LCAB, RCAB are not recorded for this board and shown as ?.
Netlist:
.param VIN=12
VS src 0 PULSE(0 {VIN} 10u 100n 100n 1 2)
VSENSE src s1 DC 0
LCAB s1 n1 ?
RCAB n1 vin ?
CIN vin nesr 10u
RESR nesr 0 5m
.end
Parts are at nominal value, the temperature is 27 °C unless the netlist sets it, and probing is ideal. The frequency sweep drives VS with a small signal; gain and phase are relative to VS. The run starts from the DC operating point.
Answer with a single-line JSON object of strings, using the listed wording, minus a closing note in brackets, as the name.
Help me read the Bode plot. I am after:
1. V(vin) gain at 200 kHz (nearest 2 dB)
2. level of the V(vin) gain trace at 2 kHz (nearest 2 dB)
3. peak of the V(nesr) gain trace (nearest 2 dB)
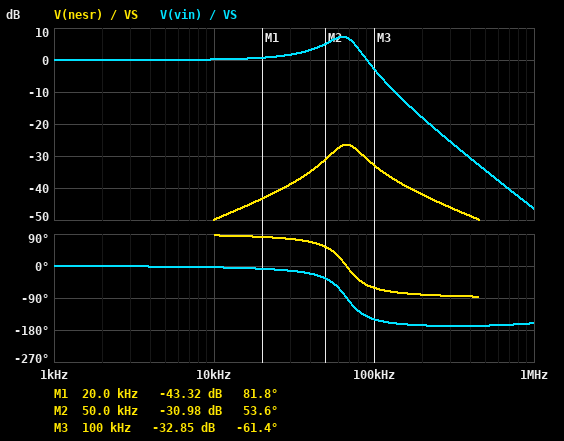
{"V(vin) gain at 200 kHz": "-18 dB", "level of the V(vin) gain trace at 2 kHz": "0 dB", "peak of the V(nesr) gain trace": "-26 dB"}
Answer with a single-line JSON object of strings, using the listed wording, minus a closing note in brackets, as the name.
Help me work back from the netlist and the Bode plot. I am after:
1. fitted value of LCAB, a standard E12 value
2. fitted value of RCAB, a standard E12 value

{"fitted value of LCAB, a standard E12 value": "560 nH", "fitted value of RCAB, a standard E12 value": "0.1 Ω"}
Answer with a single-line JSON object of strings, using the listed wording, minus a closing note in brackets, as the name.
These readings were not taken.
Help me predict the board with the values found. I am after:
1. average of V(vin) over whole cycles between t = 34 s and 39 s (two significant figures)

{"average of V(vin) over whole cycles between t = 34 s and 39 s": "6.0 V"}
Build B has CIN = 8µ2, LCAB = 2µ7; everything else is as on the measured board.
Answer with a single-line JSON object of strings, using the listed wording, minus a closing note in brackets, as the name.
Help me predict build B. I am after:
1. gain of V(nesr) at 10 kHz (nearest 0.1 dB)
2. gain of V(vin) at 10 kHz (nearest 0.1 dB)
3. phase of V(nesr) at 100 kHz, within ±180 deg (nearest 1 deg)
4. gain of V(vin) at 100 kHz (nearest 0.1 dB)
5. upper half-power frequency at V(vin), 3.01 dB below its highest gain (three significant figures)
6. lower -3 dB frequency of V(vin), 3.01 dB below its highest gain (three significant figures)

{"gain of V(nesr) at 10 kHz": "-51.0 dB", "gain of V(vin) at 10 kHz": "0.8 dB", "phase of V(nesr) at 100 kHz, within ±180 deg": "-86 deg", "gain of V(vin) at 100 kHz": "-17.8 dB", "upper half-power frequency at V(vin), 3.01 dB below its highest gain": "36.5 kHz", "lower -3 dB frequency of V(vin), 3.01 dB below its highest gain": "30.3 kHz"}
